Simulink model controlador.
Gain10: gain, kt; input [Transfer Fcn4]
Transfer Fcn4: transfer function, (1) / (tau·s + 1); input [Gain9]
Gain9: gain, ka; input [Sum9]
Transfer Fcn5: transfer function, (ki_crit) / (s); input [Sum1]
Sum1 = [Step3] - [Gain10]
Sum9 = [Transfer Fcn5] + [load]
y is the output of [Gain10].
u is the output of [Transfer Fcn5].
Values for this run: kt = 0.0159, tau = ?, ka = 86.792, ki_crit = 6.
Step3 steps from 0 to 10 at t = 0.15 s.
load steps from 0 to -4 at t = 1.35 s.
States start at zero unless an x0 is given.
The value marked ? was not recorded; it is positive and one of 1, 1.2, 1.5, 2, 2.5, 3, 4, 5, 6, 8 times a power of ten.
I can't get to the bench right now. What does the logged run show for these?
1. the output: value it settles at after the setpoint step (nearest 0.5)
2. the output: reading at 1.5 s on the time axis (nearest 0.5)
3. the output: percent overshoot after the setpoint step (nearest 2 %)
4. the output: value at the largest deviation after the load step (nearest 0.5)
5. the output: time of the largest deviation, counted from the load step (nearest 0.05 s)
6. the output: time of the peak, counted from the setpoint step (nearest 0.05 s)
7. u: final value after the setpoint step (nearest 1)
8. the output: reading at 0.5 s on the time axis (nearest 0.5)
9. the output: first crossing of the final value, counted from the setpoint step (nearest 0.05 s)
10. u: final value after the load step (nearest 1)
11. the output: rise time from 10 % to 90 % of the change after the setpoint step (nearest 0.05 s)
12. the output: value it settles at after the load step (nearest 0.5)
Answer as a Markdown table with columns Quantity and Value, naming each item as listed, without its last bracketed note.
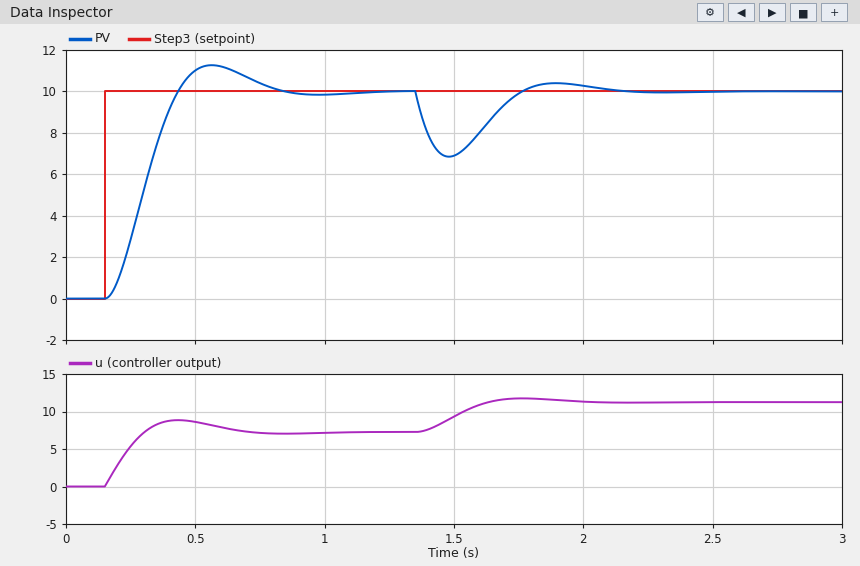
| Quantity | Value |
|---|---|
| the output: value it settles at after the setpoint step | 10.0 |
| the output: reading at 1.5 s on the time axis | 7.0 |
| the output: percent overshoot after the setpoint step | 12 % |
| the output: value at the largest deviation after the load step | 7.0 |
| the output: time of the largest deviation, counted from the load step | 0.15 s |
| the output: time of the peak, counted from the setpoint step | 0.40 s |
| u: final value after the setpoint step | 7 |
| the output: reading at 0.5 s on the time axis | 11.0 |
| the output: first crossing of the final value, counted from the setpoint step | 0.30 s |
| u: final value after the load step | 11 |
| the output: rise time from 10 % to 90 % of the change after the setpoint step | 0.20 s |
| the output: value it settles at after the load step | 10.0 |
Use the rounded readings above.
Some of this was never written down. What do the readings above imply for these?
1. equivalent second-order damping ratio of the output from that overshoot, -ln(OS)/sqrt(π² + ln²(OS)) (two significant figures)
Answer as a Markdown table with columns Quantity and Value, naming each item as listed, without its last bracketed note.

| Quantity | Value |
|---|---|
| equivalent second-order damping ratio of the output from that overshoot, -ln(OS)/sqrt(π² + ln²(OS)) | 0.56 |
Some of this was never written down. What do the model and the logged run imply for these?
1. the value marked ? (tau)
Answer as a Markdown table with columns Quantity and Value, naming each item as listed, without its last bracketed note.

| Quantity | Value |
|---|---|
| the value marked ? | 0.1 |
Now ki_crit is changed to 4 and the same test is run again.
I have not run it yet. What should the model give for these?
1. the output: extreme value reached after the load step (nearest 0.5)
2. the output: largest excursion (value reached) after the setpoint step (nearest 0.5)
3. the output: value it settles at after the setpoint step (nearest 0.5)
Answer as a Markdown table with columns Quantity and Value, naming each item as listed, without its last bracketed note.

| Quantity | Value |
|---|---|
| the output: extreme value reached after the load step | 6.5 |
| the output: largest excursion (value reached) after the setpoint step | 10.5 |
| the output: value it settles at after the setpoint step | 10.0 |
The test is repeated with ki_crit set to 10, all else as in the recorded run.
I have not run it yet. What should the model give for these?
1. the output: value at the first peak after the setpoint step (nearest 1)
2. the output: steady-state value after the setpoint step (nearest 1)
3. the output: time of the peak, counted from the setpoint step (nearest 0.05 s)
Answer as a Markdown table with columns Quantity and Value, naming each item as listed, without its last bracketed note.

| Quantity | Value |
|---|---|
| the output: value at the first peak after the setpoint step | 12 |
| the output: steady-state value after the setpoint step | 10 |
| the output: time of the peak, counted from the setpoint step | 0.30 s |
